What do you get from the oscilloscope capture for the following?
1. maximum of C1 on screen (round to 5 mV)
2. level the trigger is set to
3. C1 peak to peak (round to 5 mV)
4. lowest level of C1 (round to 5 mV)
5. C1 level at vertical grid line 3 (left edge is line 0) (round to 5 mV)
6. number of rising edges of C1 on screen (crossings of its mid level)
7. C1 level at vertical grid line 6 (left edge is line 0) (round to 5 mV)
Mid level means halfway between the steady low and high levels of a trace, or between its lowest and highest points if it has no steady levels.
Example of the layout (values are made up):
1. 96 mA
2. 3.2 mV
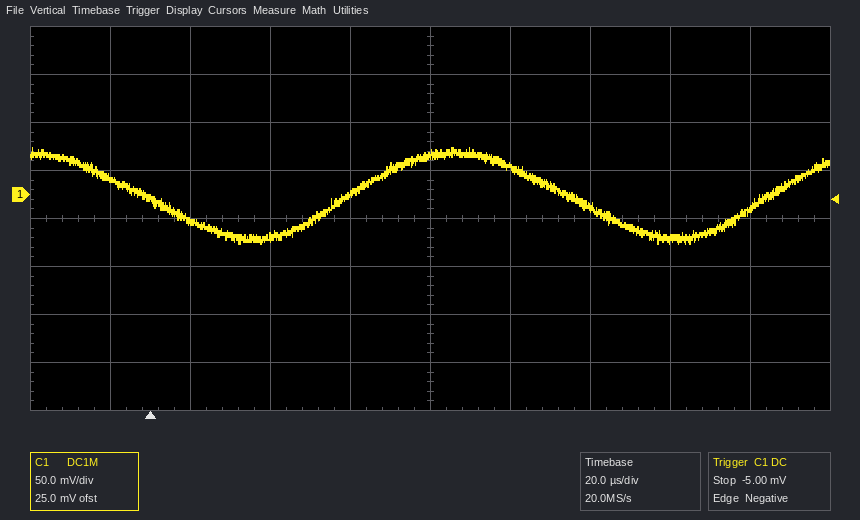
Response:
1. 50 mV
2. -5.00 mV
3. 100 mV
4. -50 mV
5. -45 mV
6. 2
7. 30 mV
